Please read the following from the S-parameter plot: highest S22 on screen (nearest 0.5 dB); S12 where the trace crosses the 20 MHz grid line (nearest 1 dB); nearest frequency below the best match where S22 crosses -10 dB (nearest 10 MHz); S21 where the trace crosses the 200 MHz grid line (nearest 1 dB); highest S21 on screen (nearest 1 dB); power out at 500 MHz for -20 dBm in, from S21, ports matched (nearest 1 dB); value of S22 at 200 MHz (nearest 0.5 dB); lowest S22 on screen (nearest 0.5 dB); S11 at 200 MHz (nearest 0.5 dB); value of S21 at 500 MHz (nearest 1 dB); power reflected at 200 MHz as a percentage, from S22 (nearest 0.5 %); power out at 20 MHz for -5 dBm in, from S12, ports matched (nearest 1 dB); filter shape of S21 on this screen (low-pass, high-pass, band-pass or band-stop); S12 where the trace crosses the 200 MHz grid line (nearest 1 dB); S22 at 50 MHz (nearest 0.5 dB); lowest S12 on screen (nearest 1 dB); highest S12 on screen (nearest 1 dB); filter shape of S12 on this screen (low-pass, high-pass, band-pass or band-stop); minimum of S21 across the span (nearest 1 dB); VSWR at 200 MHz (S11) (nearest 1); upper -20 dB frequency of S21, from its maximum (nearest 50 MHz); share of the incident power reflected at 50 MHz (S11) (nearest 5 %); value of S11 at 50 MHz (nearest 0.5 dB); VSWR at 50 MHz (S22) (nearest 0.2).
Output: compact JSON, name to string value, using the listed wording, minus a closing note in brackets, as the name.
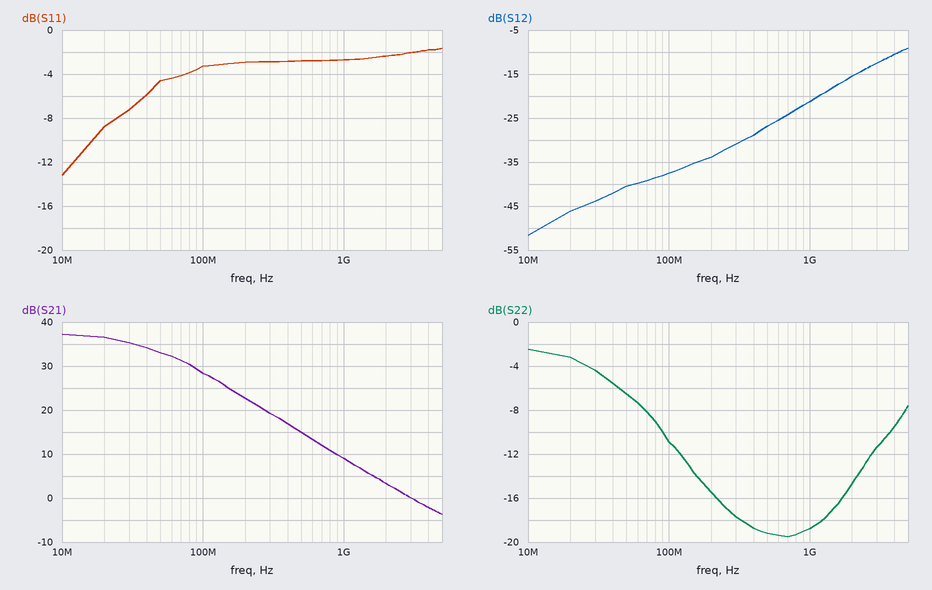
{"highest S22 on screen": "-2.5 dB", "S12 where the trace crosses the 20 MHz grid line": "-46 dB", "nearest frequency below the best match where S22 crosses -10 dB": "90 MHz", "S21 where the trace crosses the 200 MHz grid line": "23 dB", "highest S21 on screen": "37 dB", "power out at 500 MHz for -20 dBm in, from S21, ports matched": "-5 dBm", "value of S22 at 200 MHz": "-15.5 dB", "lowest S22 on screen": "-19.5 dB", "S11 at 200 MHz": "-3.0 dB", "value of S21 at 500 MHz": "15 dB", "power reflected at 200 MHz as a percentage, from S22": "3.0 %", "power out at 20 MHz for -5 dBm in, from S12, ports matched": "-51 dBm", "filter shape of S21 on this screen": "low-pass", "S12 where the trace crosses the 200 MHz grid line": "-34 dB", "S22 at 50 MHz": "-6.5 dB", "lowest S12 on screen": "-52 dB", "highest S12 on screen": "-9 dB", "filter shape of S12 on this screen": "high-pass", "minimum of S21 across the span": "-4 dB", "VSWR at 200 MHz (S11)": "6", "upper -20 dB frequency of S21, from its maximum": "400 MHz", "share of the incident power reflected at 50 MHz (S11)": "35 %", "value of S11 at 50 MHz": "-4.5 dB", "VSWR at 50 MHz (S22)": "2.8"}
